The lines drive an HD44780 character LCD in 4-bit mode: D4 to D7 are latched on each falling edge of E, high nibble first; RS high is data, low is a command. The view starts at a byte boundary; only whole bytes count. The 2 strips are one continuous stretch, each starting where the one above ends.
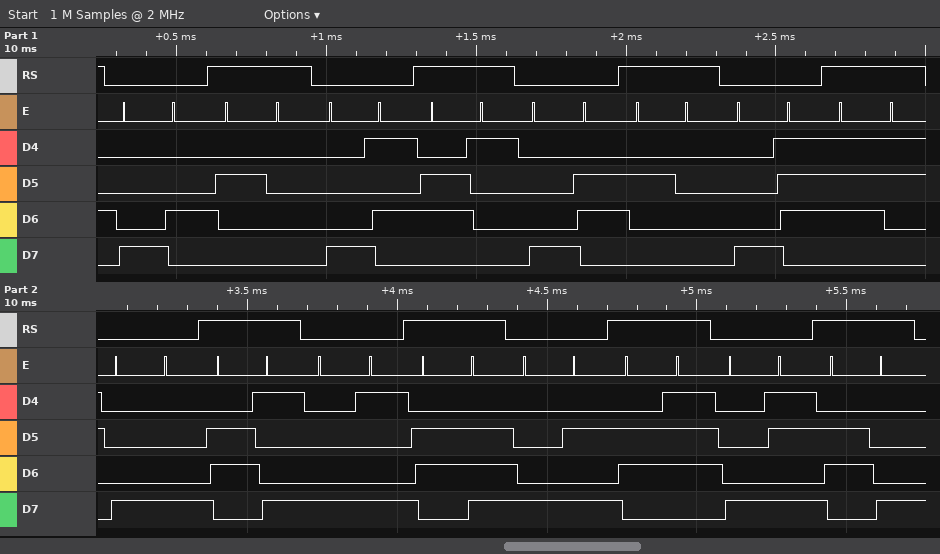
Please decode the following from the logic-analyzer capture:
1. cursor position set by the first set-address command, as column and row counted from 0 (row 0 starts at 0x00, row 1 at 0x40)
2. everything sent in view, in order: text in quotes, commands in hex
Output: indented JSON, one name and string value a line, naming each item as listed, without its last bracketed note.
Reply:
{
  "cursor position set by the first set-address command, as column and row counted from 0": "column 4, row 0",
  "everything sent in view, in order: text in quotes, commands in hex": "0x84 \" \" 0x85 \"a\" 0x86 \" \" 0x87 \"s\" 0x88 \"i\" 0x89 \"n\" 0x8A \"g\" 0x8B \"h\""
}
